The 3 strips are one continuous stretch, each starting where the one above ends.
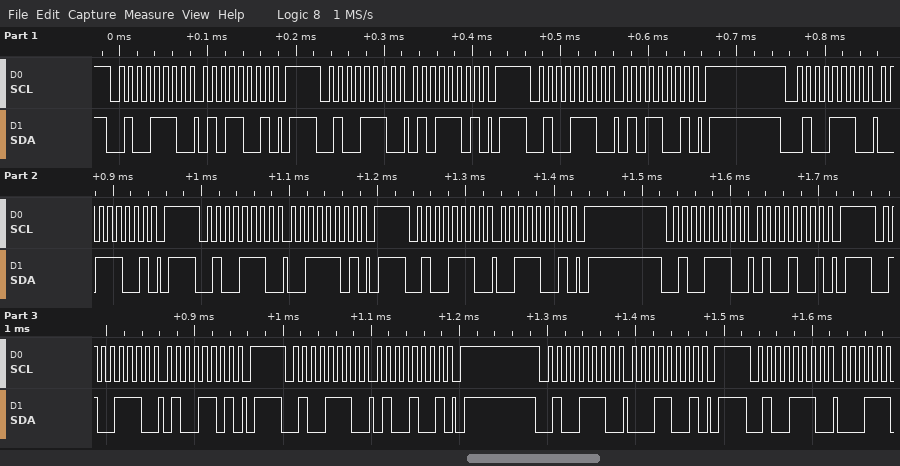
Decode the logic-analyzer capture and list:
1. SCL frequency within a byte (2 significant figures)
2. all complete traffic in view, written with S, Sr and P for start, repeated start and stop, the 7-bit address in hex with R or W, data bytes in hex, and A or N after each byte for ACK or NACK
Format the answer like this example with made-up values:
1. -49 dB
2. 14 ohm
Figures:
1. 100 kHz
2. S 27W A 59 A P S 27W A 5D A P S 27W A 59 A P S 27W A 39 A P S 27W A 3D A P S 27W A 39 A P S 27W A 49 A P S 27W A 4D A P S 27W A 49 A P S 27W A 19 A P S 27W A
